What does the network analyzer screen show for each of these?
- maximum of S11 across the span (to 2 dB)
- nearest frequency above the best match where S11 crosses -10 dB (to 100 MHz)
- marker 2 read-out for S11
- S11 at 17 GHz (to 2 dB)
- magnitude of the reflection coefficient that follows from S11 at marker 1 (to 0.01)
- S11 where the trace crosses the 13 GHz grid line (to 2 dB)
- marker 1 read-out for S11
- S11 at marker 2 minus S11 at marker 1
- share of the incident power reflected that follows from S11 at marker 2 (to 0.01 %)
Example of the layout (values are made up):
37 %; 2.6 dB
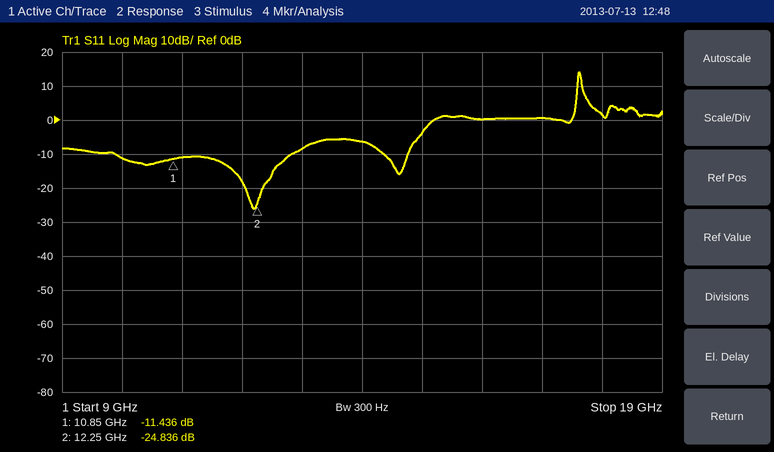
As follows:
14 dB; 12.8 GHz; -24.836 dB; 0 dB; 0.27; -8 dB; -11.436 dB; -13.400 dB; 0.33 %
